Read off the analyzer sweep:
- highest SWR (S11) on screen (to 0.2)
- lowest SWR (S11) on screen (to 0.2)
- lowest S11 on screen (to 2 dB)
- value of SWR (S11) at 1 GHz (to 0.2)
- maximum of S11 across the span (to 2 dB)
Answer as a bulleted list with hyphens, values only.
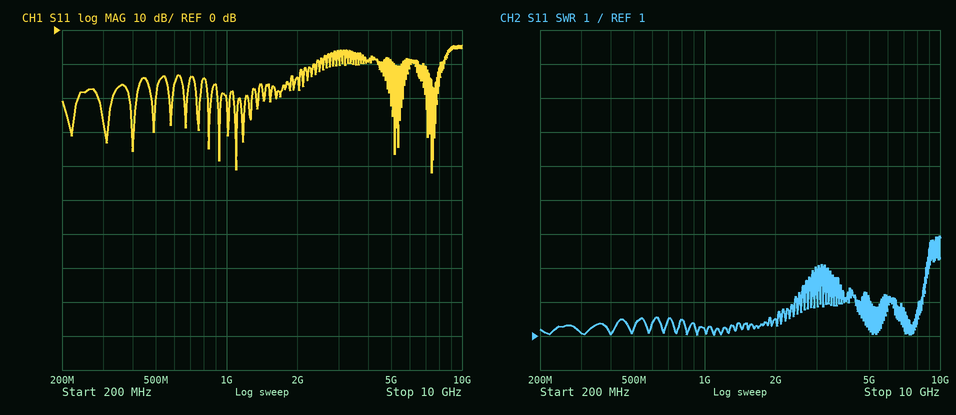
- 4.0
- 1.0
- -42 dB
- 1.2
- -4 dB
